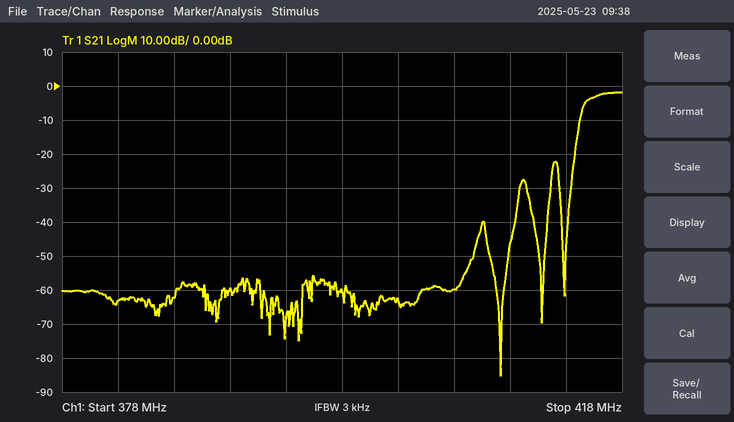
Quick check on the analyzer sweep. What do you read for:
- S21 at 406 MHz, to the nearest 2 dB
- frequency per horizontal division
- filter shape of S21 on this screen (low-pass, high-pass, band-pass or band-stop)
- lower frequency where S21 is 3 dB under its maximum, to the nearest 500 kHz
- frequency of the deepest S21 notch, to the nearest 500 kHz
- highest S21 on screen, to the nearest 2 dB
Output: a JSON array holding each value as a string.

["-60 dB", "4 MHz", "high-pass", "415.5 MHz", "409.5 MHz", "-2 dB"]
